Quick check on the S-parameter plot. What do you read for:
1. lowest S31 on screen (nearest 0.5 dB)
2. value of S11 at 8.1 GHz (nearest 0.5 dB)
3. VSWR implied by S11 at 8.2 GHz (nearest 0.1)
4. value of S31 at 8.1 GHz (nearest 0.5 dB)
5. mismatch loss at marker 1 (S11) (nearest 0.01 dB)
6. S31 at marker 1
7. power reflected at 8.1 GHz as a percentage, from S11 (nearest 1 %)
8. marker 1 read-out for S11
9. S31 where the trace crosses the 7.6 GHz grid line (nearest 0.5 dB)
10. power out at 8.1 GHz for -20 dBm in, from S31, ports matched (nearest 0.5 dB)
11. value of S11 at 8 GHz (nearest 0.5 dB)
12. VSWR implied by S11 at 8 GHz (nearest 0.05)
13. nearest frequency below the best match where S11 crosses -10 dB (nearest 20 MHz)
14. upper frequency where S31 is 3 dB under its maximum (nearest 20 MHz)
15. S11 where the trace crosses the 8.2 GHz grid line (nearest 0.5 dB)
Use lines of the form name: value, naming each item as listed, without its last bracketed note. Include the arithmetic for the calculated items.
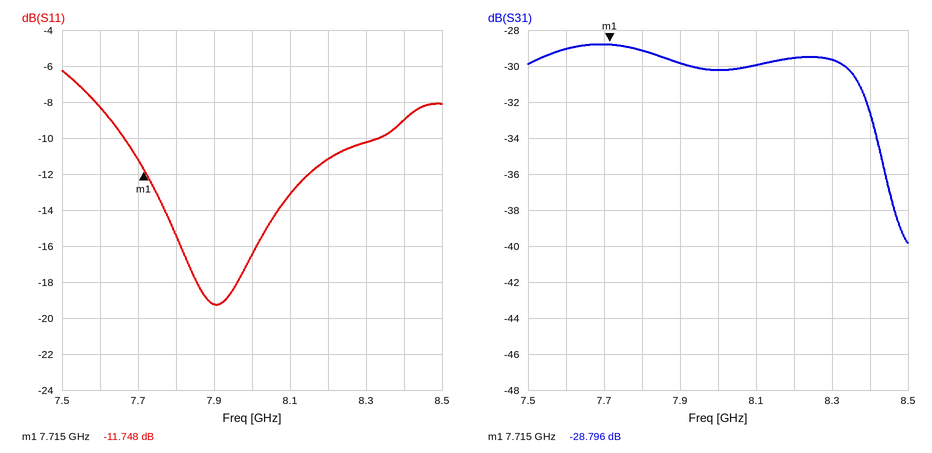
lowest S31 on screen: -40.0 dB
value of S11 at 8.1 GHz: -13.0 dB
VSWR implied by S11 at 8.2 GHz: |Γ| = 10^(-11/20) = 0.2818; VSWR = (1 + 0.2818)/(1 − 0.2818) ≈ 1.8
value of S31 at 8.1 GHz: -30.0 dB
mismatch loss at marker 1 (S11): −10 log10(1 − 10^(-11.748/10)) ≈ 0.30 dB
S31 at marker 1: -28.796 dB
power reflected at 8.1 GHz as a percentage, from S11: 10^(-13/10) ≈ 5 %
marker 1 read-out for S11: -11.748 dB
S31 where the trace crosses the 7.6 GHz grid line: -29.0 dB
power out at 8.1 GHz for -20 dBm in, from S31, ports matched: -20 dBm + (-30.0 dB) = -50.0 dBm
value of S11 at 8 GHz: -16.5 dB
VSWR implied by S11 at 8 GHz: |Γ| = 10^(-16.5/20) = 0.1496; VSWR = (1 + 0.1496)/(1 − 0.1496) ≈ 1.35
nearest frequency below the best match where S11 crosses -10 dB: 7.66 GHz
upper frequency where S31 is 3 dB under its maximum: 8.38 GHz
S11 where the trace crosses the 8.2 GHz grid line: -11.0 dB
